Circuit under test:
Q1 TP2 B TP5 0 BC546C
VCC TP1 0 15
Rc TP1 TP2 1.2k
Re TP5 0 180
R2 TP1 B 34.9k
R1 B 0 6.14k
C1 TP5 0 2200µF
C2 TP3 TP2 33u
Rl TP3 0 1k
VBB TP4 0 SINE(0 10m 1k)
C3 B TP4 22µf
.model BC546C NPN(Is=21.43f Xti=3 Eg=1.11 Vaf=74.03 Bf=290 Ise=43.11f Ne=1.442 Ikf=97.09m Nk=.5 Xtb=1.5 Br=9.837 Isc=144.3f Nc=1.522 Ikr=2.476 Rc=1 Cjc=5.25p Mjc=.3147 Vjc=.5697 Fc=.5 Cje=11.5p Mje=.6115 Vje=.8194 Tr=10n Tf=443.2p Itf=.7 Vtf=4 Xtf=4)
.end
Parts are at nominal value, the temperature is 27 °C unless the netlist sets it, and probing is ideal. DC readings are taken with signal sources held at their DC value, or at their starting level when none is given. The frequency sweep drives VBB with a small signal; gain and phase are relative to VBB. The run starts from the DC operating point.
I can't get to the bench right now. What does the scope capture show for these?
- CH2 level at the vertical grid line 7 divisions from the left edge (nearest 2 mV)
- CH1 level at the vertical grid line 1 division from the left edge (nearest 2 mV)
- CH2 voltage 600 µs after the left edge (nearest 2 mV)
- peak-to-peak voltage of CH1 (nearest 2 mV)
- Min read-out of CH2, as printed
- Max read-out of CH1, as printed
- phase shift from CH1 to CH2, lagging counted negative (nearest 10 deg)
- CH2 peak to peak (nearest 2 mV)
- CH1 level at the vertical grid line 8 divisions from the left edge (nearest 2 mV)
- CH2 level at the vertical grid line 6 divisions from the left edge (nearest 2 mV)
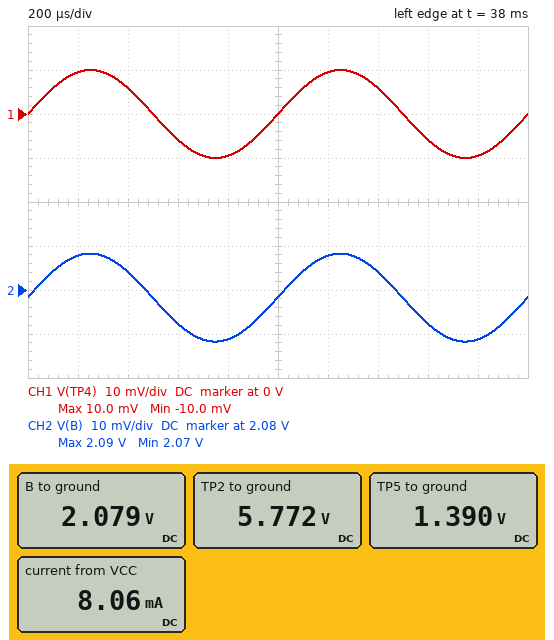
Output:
2.084 V
10 mV
2.072 V
20 mV
2.07 V
10.0 mV
0 deg
20 mV
-6 mV
2.088 V
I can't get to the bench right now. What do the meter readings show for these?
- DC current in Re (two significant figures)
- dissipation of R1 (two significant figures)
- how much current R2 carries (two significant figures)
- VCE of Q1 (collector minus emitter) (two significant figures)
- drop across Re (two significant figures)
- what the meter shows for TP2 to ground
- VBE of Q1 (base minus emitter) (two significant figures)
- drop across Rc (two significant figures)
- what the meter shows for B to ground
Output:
7.7 mA
700 µW
370 µA
4.4 V
1.4 V
5.772 V
690 mV
9.2 V
2.079 V
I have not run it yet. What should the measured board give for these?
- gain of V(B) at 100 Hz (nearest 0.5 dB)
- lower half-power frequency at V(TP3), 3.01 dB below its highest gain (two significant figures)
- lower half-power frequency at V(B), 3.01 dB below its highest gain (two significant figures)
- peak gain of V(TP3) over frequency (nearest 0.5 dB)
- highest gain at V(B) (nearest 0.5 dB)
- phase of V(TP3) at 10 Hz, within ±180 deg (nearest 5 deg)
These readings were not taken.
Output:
0 dB
29 Hz
7.4 Hz
43.0 dB
0 dB
-95 deg
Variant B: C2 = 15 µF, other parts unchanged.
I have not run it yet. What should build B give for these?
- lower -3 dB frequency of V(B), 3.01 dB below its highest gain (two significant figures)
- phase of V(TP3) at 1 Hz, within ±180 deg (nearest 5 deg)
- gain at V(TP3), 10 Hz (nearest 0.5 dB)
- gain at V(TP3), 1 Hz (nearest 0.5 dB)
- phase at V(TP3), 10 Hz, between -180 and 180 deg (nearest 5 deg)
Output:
7.5 Hz
10 deg
32.5 dB
-2.5 dB
-80 deg
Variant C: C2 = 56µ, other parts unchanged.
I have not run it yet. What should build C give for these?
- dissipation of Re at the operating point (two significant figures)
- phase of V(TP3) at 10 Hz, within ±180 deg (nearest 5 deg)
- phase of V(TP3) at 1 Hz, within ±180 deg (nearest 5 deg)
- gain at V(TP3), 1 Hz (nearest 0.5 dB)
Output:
11 mW
-100 deg
-15 deg
7.0 dB
